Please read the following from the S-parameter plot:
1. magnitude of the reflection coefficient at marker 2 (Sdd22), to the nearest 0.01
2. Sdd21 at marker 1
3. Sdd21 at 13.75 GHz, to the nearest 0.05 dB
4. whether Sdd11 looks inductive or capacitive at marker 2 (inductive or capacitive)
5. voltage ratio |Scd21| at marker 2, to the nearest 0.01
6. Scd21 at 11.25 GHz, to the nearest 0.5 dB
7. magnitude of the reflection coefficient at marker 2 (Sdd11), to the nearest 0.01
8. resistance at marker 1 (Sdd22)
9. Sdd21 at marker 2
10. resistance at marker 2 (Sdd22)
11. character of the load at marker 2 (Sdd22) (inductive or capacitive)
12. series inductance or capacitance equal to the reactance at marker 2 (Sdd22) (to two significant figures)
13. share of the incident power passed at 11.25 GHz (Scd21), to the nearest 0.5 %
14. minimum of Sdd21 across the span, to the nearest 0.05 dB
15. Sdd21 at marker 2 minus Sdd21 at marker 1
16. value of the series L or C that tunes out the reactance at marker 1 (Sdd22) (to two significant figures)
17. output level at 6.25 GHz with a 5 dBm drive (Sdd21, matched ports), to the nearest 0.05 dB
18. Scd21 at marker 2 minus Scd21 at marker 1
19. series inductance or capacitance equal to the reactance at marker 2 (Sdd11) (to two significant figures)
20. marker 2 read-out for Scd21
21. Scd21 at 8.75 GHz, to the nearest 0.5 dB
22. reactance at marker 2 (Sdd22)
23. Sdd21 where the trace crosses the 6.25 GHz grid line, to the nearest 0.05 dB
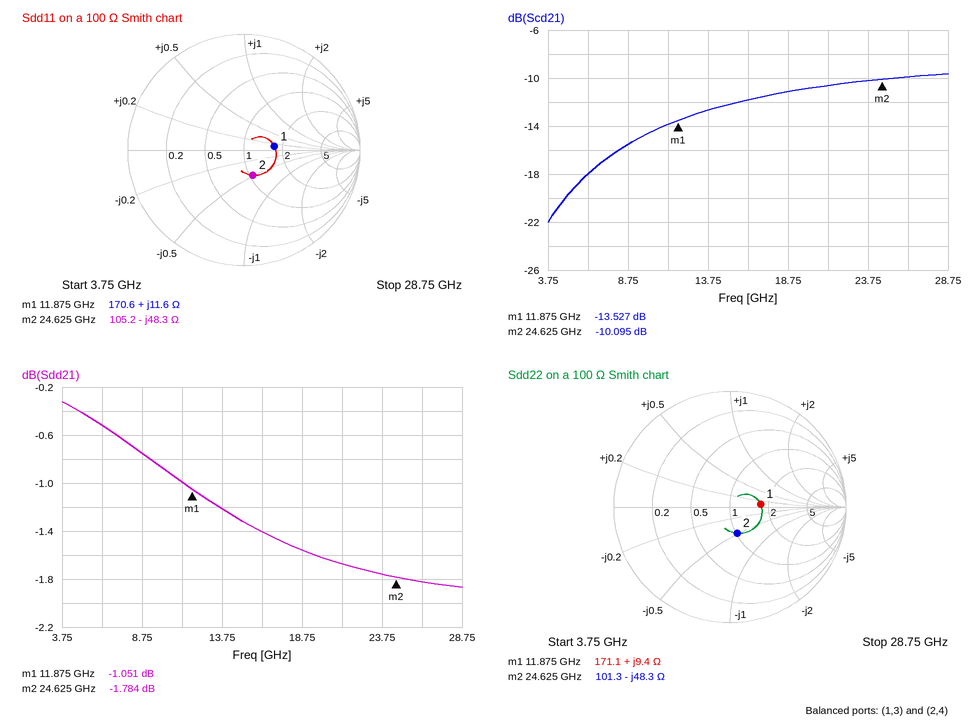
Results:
0.23
-1.051 dB
-1.20 dB
capacitive
0.31
-14.0 dB
0.23
171.1 Ω
-1.784 dB
101.3 Ω
capacitive
130 fF
4.0 %
-1.85 dB
-0.733 dB
1.4 pF
4.50 dBm
3.432 dB
130 fF
-10.095 dB
-15.5 dB
-48.3 Ω
-0.50 dB
